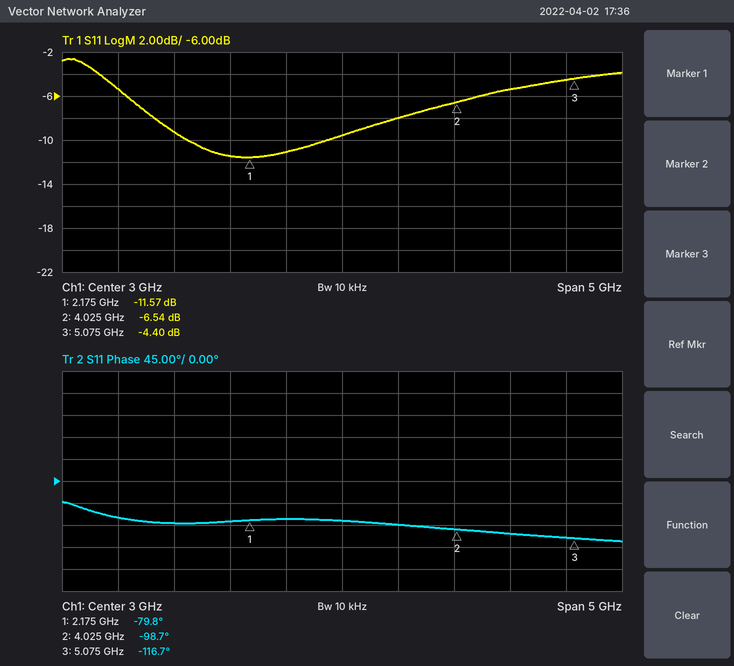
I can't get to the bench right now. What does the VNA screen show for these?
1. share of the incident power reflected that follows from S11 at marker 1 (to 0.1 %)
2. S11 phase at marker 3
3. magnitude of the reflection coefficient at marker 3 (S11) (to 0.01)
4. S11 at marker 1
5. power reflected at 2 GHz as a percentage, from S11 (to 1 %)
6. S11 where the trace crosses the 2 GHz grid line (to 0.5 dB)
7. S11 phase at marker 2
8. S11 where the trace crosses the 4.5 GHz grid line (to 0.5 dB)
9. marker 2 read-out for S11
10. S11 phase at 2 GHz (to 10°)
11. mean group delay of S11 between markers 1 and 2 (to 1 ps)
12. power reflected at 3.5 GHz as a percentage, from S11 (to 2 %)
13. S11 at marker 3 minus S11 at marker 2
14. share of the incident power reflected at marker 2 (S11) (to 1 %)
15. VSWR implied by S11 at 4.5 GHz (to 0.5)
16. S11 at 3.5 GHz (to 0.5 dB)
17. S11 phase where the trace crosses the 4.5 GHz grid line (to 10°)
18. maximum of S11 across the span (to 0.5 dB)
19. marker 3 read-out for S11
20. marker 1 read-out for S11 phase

7.0 %
-116.7°
0.60
-11.57 dB
7 %
-11.5 dB
-98.7°
-5.5 dB
-6.54 dB
-80°
28 ps
16 %
2.14 dB
22 %
3.5
-8.0 dB
-110°
-2.5 dB
-4.40 dB
-79.8°
